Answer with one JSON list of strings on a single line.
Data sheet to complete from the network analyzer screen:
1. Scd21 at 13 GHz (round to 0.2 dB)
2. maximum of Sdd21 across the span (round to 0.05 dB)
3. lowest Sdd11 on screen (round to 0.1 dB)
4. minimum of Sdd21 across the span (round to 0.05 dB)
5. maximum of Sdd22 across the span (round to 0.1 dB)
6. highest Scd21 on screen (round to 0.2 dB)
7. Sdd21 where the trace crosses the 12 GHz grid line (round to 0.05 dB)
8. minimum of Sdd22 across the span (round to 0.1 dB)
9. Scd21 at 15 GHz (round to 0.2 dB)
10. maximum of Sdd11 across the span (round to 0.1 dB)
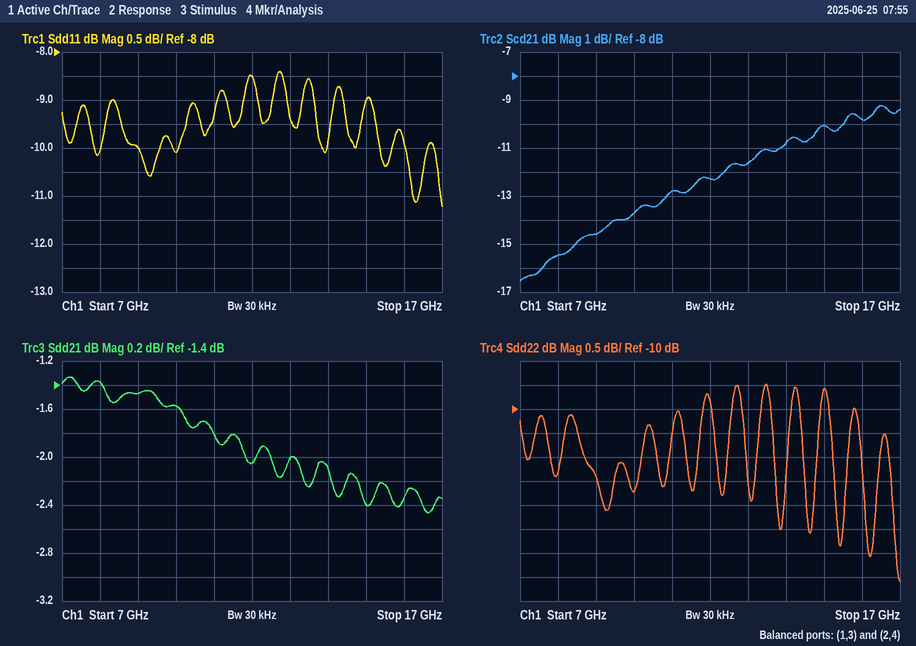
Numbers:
["-11.6 dB", "-1.35 dB", "-11.2 dB", "-2.45 dB", "-9.5 dB", "-9.2 dB", "-2.05 dB", "-13.6 dB", "-10.0 dB", "-8.4 dB"]
